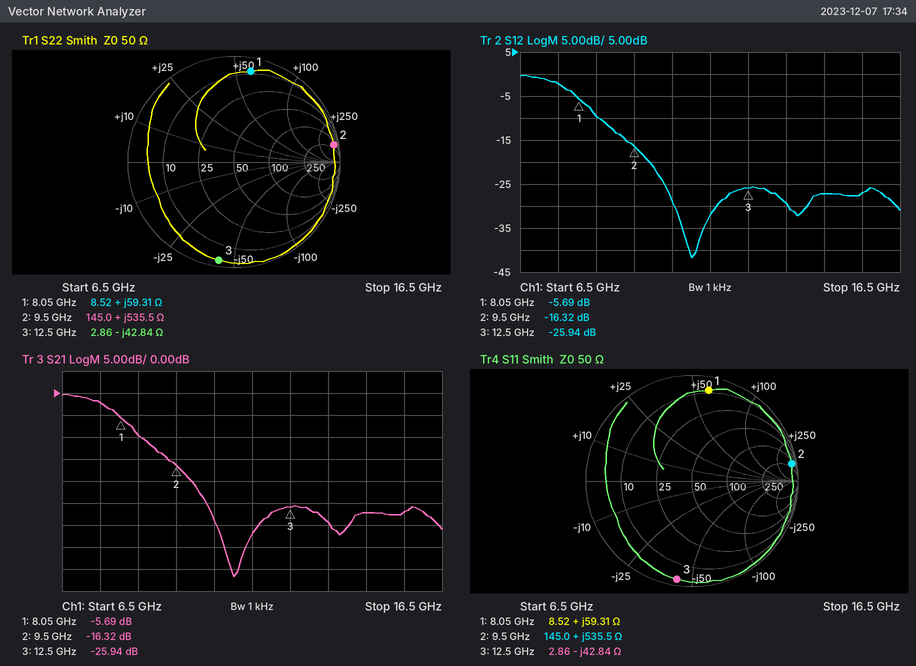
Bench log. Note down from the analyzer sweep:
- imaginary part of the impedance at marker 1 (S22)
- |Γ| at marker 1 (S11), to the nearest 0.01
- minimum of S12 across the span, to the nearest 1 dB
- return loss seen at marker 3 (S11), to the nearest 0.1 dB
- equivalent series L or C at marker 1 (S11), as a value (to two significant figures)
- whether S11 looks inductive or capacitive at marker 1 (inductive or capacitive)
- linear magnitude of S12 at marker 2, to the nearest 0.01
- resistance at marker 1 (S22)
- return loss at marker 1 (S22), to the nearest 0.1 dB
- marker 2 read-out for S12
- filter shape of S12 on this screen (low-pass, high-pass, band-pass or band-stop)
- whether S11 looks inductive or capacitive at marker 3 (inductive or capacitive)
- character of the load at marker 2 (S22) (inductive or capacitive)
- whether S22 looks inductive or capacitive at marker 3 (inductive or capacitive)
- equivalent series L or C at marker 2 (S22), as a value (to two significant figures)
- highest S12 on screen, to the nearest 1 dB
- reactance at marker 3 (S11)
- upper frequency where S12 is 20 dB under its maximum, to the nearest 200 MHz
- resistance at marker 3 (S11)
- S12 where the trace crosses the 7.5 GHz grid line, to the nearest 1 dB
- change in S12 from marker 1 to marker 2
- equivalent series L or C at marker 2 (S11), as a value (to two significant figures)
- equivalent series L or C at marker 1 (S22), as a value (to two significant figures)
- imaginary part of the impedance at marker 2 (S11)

+59.31 Ω
0.87
-42 dB
0.6 dB
1.2 nH
inductive
0.15
8.52 Ω
1.2 dB
-16.32 dB
low-pass
capacitive
inductive
capacitive
9.0 nH
0 dB
-42.84 Ω
10.0 GHz
2.86 Ω
-2 dB
-10.63 dB
9.0 nH
1.2 nH
+535.5 Ω
